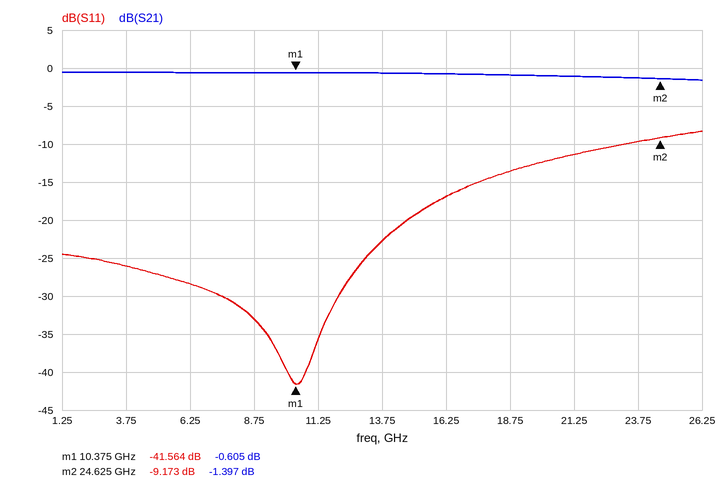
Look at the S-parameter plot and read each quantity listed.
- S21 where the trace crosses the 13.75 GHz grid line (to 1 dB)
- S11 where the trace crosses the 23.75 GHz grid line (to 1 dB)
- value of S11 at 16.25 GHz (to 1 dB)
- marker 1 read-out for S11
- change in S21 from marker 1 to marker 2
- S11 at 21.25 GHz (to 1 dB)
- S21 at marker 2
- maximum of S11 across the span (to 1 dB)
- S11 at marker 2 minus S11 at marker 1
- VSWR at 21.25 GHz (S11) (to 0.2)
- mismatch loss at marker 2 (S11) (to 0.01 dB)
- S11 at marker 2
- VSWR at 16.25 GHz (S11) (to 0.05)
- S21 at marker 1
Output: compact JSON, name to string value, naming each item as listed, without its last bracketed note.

{"S21 where the trace crosses the 13.75 GHz grid line": "-1 dB", "S11 where the trace crosses the 23.75 GHz grid line": "-10 dB", "value of S11 at 16.25 GHz": "-17 dB", "marker 1 read-out for S11": "-41.564 dB", "change in S21 from marker 1 to marker 2": "-0.792 dB", "S11 at 21.25 GHz": "-11 dB", "S21 at marker 2": "-1.397 dB", "maximum of S11 across the span": "-8 dB", "S11 at marker 2 minus S11 at marker 1": "32.391 dB", "VSWR at 21.25 GHz (S11)": "1.8", "mismatch loss at marker 2 (S11)": "0.56 dB", "S11 at marker 2": "-9.173 dB", "VSWR at 16.25 GHz (S11)": "1.35", "S21 at marker 1": "-0.605 dB"}
